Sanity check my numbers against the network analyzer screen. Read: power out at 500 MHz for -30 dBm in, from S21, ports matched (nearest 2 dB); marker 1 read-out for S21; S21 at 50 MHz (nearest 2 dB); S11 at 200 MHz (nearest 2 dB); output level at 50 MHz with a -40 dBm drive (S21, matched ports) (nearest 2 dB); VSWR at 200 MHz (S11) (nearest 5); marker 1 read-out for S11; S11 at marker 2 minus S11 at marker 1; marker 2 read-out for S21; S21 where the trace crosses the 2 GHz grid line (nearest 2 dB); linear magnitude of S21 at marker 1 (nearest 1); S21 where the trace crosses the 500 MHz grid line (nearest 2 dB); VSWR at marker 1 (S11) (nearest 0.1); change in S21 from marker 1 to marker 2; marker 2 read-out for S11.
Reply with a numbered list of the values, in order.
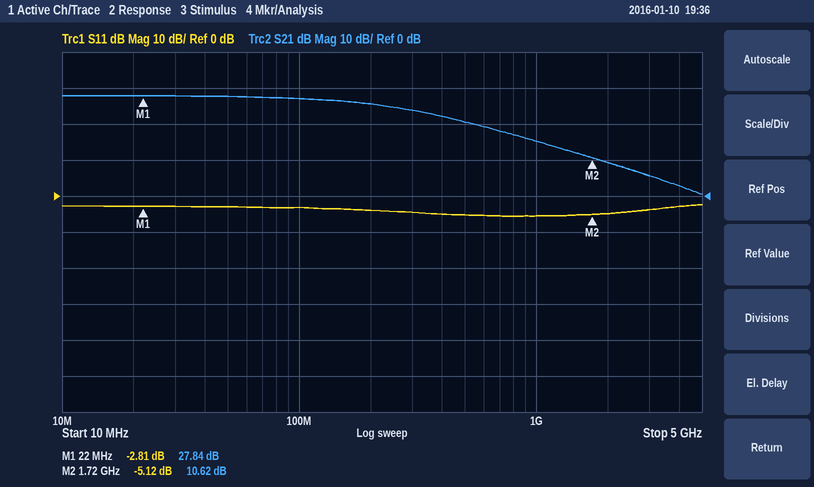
1. -10 dBm
2. 27.84 dB
3. 28 dB
4. -4 dB
5. -12 dBm
6. 5
7. -2.81 dB
8. -2.31 dB
9. 10.62 dB
10. 10 dB
11. 25
12. 20 dB
13. 6.2
14. -17.22 dB
15. -5.12 dB
